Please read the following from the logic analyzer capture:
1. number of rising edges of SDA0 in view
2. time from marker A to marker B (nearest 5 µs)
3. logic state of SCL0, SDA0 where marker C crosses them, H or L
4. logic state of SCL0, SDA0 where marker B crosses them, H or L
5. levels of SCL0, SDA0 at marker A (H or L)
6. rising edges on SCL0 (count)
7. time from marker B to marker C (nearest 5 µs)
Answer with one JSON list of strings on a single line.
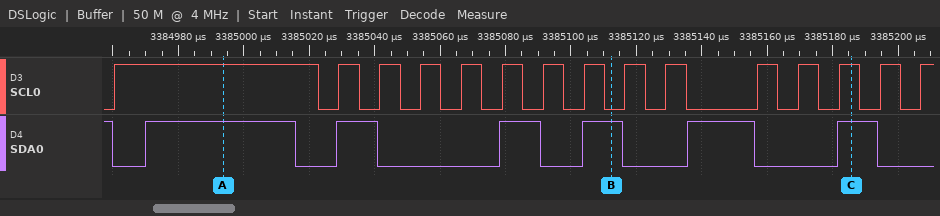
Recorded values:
["6", "120 µs", "SCL0=H, SDA0=H", "SCL0=L, SDA0=H", "SCL0=H, SDA0=H", "15", "75 µs"]
